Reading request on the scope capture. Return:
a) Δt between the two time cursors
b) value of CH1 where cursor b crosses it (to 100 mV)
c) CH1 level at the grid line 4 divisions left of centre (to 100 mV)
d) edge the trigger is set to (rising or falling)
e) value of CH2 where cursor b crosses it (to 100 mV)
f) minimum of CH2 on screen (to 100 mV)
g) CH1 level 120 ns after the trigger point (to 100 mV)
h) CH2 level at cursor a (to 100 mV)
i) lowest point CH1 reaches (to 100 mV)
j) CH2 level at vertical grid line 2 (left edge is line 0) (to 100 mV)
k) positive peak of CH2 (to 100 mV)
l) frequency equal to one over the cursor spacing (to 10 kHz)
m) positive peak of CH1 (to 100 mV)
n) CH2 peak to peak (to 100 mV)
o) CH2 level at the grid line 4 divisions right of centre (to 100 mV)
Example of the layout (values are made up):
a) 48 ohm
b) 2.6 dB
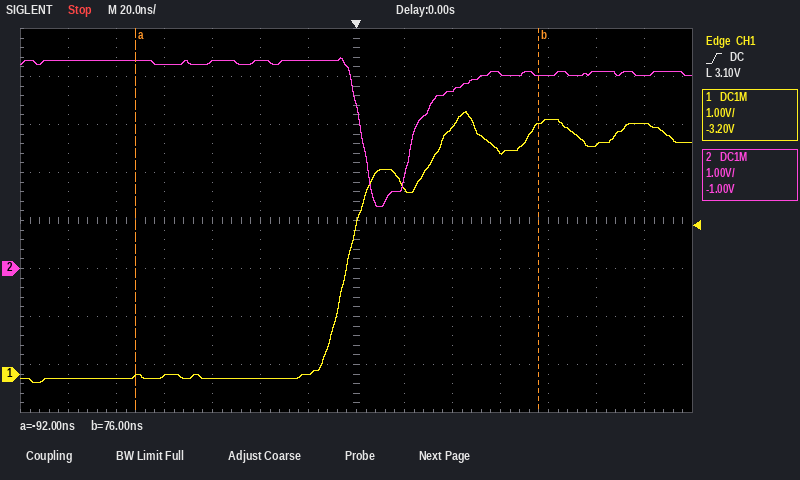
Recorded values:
a) 168 ns
b) 5.2 V
c) 0.0 V
d) rising
e) 4.0 V
f) 1.3 V
g) 5.2 V
h) 4.3 V
i) -200 mV
j) 4.3 V
k) 4.4 V
l) 5.95 MHz
m) 5.5 V
n) 3.1 V
o) 4.0 V
